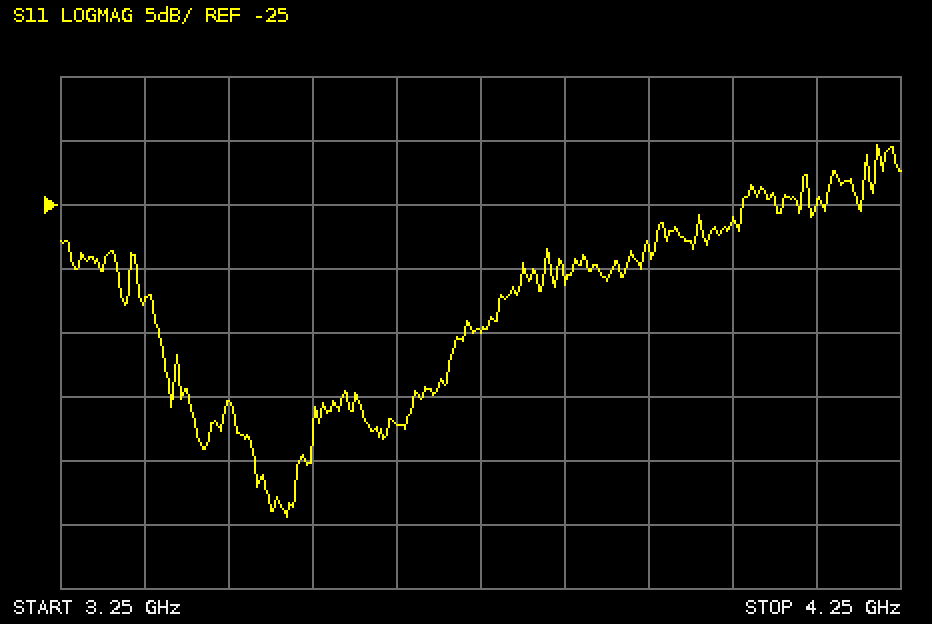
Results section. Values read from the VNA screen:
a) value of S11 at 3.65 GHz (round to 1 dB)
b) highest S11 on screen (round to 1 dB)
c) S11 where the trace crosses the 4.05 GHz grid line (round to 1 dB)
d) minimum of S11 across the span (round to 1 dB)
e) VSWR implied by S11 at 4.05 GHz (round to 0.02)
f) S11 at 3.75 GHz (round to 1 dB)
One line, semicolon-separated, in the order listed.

-42 dB; -20 dB; -26 dB; -49 dB; 1.10; -35 dB
